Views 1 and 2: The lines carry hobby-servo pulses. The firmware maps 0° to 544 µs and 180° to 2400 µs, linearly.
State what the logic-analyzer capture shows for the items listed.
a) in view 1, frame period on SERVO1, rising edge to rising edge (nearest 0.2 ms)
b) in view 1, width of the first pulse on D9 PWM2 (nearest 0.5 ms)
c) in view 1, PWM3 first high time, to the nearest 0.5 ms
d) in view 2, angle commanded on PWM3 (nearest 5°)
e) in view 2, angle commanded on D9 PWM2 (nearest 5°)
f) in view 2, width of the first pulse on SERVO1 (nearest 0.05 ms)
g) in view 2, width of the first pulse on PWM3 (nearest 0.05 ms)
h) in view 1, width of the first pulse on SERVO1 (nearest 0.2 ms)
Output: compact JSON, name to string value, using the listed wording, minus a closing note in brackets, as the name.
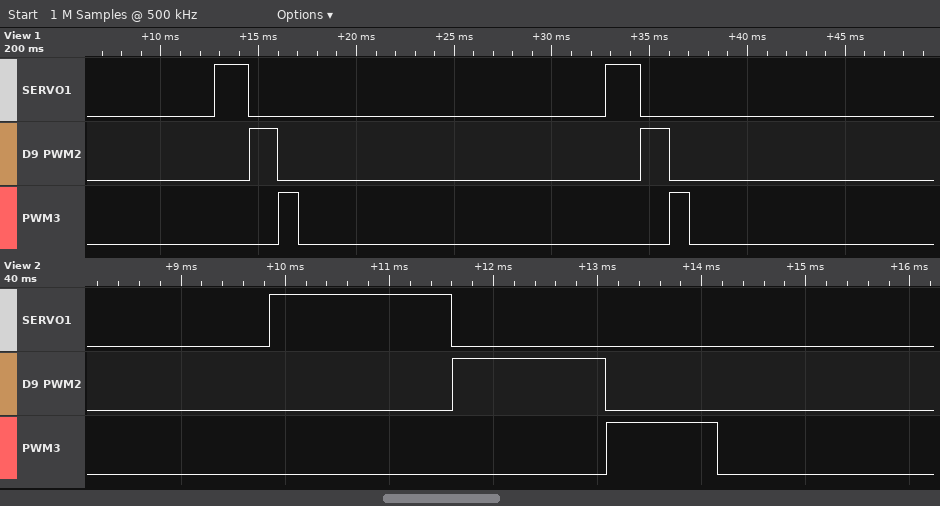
{"in view 1, frame period on SERVO1, rising edge to rising edge": "20.0 ms", "in view 1, width of the first pulse on D9 PWM2": "1.5 ms", "in view 1, PWM3 first high time, to the nearest 0.5 ms": "1.0 ms", "in view 2, angle commanded on PWM3": "50°", "in view 2, angle commanded on D9 PWM2": "90°", "in view 2, width of the first pulse on SERVO1": "1.75 ms", "in view 2, width of the first pulse on PWM3": "1.05 ms", "in view 1, width of the first pulse on SERVO1": "1.8 ms"}
